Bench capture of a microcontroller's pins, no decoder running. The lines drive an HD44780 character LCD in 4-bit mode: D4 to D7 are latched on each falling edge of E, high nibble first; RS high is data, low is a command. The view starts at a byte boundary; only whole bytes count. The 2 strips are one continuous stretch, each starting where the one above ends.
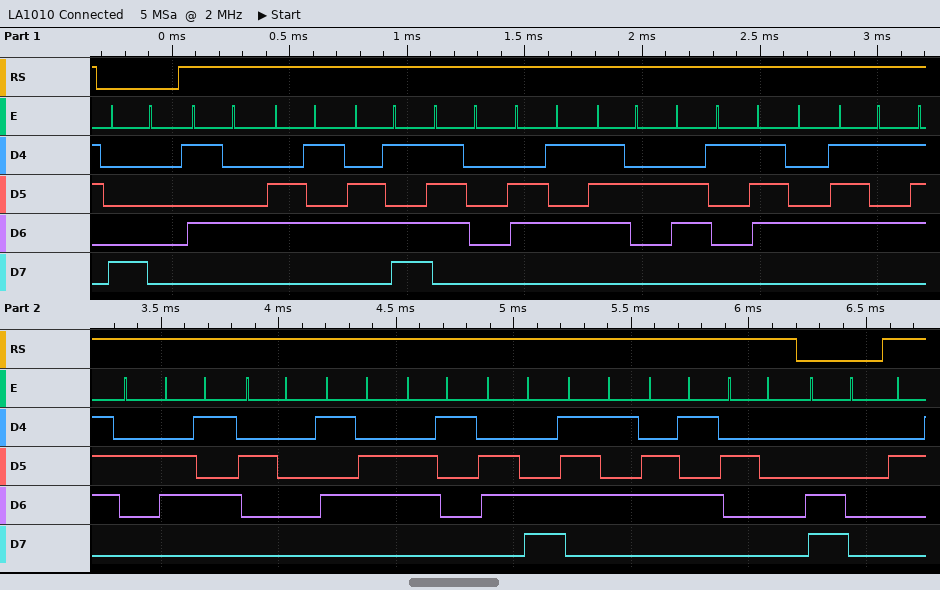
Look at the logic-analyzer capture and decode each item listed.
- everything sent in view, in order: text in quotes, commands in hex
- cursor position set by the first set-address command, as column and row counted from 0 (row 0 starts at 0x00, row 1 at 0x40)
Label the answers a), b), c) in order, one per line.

a) 0x80 "Temperature Value " 0xC0
b) column 0, row 0
